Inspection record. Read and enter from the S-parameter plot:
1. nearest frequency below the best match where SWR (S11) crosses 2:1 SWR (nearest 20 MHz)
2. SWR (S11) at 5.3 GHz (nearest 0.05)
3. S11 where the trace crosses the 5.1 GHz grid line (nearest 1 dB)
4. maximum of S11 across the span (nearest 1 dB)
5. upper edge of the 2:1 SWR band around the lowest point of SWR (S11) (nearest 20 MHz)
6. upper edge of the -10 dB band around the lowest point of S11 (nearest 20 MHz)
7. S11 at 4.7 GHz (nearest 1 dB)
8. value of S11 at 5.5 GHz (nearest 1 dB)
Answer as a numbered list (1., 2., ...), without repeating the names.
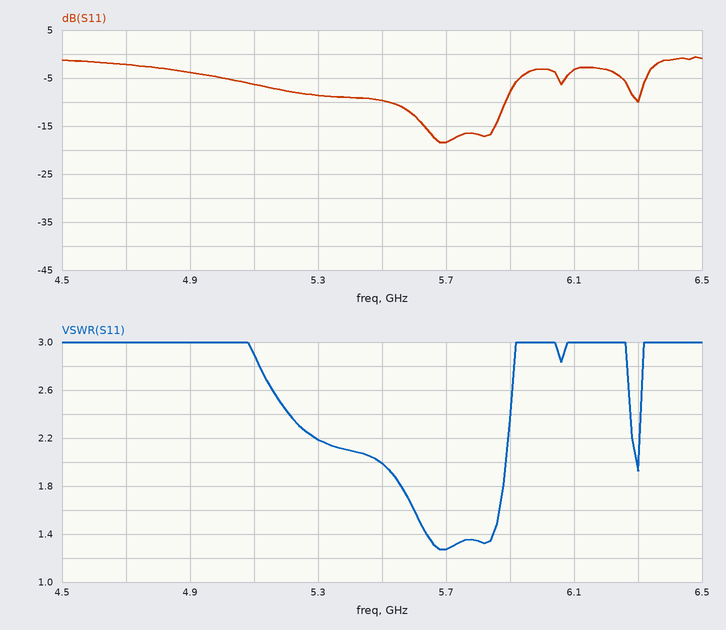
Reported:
1. 5.50 GHz
2. 2.20
3. -6 dB
4. -1 dB
5. 5.88 GHz
6. 5.88 GHz
7. -2 dB
8. -10 dB
